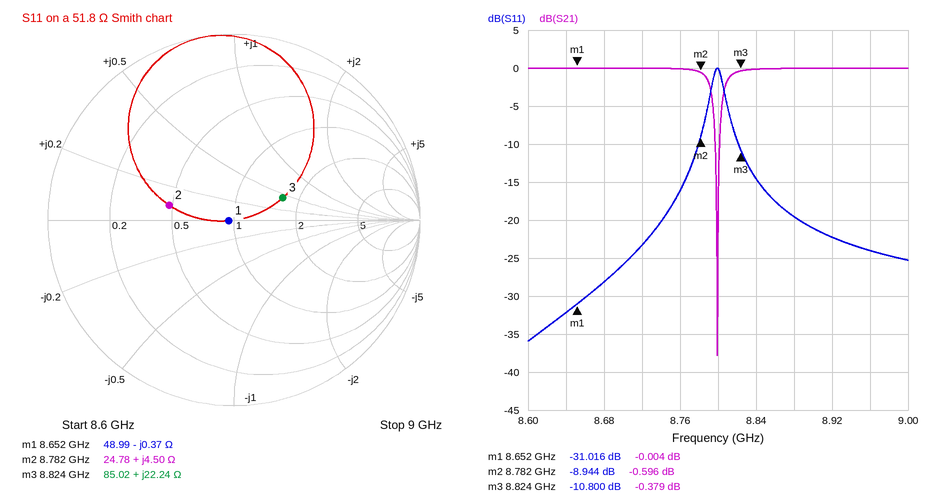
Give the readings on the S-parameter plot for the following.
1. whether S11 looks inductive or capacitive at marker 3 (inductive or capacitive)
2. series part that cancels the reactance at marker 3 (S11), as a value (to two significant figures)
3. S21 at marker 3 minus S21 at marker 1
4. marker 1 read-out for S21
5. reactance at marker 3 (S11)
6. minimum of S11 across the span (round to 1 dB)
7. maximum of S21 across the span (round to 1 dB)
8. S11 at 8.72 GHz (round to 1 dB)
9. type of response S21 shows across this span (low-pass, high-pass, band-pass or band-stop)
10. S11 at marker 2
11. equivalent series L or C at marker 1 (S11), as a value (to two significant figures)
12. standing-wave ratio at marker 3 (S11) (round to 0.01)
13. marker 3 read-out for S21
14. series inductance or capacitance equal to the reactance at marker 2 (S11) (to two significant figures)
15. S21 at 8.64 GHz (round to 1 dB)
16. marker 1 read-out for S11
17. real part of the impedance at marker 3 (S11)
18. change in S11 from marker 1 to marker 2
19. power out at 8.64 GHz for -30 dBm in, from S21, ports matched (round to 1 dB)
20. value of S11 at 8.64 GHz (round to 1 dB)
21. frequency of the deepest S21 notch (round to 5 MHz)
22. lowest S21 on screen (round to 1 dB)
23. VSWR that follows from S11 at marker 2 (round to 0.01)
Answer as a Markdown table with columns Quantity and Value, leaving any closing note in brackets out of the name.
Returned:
| Quantity | Value |
|---|---|
| whether S11 looks inductive or capacitive at marker 3 | inductive |
| series part that cancels the reactance at marker 3 (S11), as a value | 810 fF |
| S21 at marker 3 minus S21 at marker 1 | -0.375 dB |
| marker 1 read-out for S21 | -0.004 dB |
| reactance at marker 3 | +22.24 Ω |
| minimum of S11 across the span | -36 dB |
| maximum of S21 across the span | 0 dB |
| S11 at 8.72 GHz | -23 dB |
| type of response S21 shows across this span | band-stop |
| S11 at marker 2 | -8.944 dB |
| equivalent series L or C at marker 1 (S11), as a value | 50 pF |
| standing-wave ratio at marker 3 (S11) | 1.81 |
| marker 3 read-out for S21 | -0.379 dB |
| series inductance or capacitance equal to the reactance at marker 2 (S11) | 82 pH |
| S21 at 8.64 GHz | 0 dB |
| marker 1 read-out for S11 | -31.016 dB |
| real part of the impedance at marker 3 | 85.02 Ω |
| change in S11 from marker 1 to marker 2 | 22.072 dB |
| power out at 8.64 GHz for -30 dBm in, from S21, ports matched | -30 dBm |
| value of S11 at 8.64 GHz | -32 dB |
| frequency of the deepest S21 notch | 8.800 GHz |
| lowest S21 on screen | -38 dB |
| VSWR that follows from S11 at marker 2 | 2.11 |
